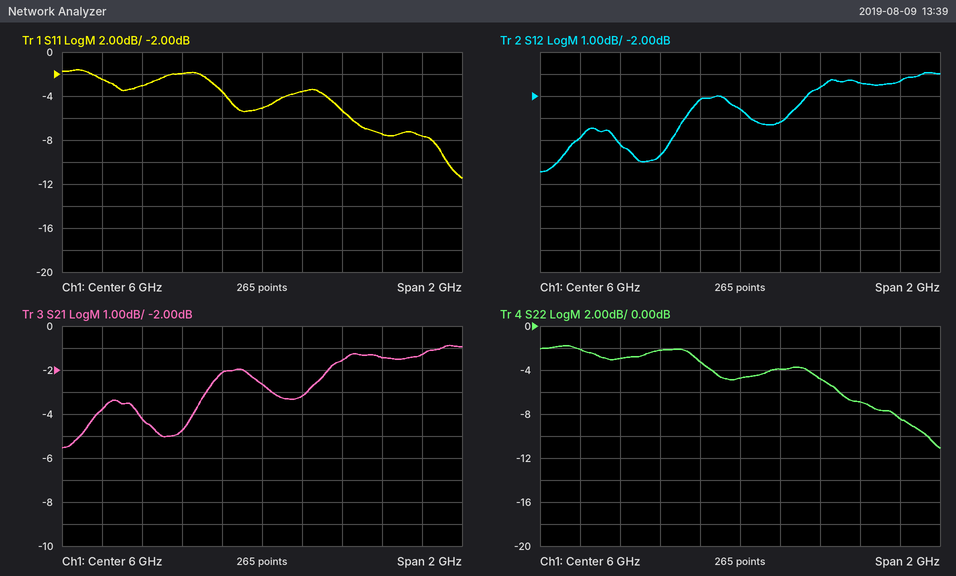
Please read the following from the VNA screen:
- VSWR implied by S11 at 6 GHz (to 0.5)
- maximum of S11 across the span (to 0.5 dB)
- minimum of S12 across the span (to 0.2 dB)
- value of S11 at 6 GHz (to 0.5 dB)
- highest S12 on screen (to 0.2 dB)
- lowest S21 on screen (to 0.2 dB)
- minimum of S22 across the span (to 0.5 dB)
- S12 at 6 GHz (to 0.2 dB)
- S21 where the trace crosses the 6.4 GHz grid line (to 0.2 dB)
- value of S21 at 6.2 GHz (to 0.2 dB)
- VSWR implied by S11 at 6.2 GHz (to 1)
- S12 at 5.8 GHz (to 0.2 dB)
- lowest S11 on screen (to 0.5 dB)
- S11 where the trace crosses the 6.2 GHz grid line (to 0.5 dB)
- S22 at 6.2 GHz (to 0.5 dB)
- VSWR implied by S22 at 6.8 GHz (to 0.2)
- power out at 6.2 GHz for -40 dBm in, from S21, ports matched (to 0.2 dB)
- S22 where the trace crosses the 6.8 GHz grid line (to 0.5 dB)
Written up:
3.5
-1.5 dB
-5.4 dB
-5.0 dB
-1.0 dB
-5.6 dB
-11.0 dB
-2.6 dB
-1.6 dB
-3.2 dB
5
-2.2 dB
-11.5 dB
-3.5 dB
-4.0 dB
2.2
-43.2 dBm
-8.5 dB
